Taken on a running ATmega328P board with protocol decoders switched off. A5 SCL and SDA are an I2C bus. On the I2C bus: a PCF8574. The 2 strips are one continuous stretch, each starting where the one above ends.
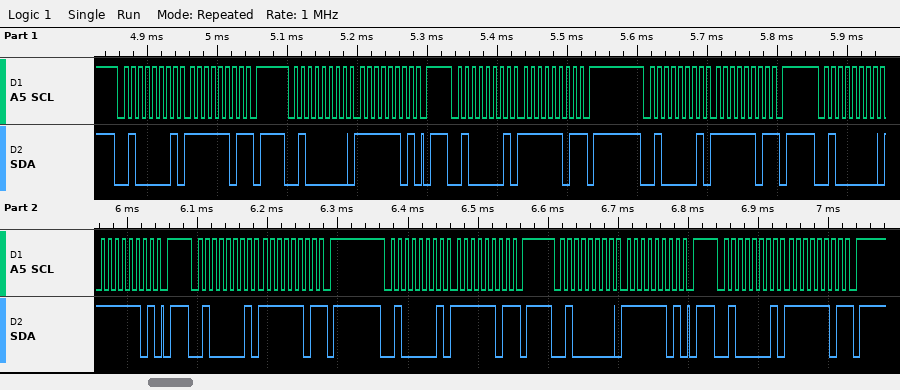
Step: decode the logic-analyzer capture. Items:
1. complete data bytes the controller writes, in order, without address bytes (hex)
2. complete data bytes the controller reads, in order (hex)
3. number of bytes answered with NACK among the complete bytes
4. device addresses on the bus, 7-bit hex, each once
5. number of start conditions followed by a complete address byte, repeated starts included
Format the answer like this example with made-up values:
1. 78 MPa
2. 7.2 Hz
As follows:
1. FD FD FD
2. FD FD FD FD FD FD
3. 6
4. 0x20
5. 9
